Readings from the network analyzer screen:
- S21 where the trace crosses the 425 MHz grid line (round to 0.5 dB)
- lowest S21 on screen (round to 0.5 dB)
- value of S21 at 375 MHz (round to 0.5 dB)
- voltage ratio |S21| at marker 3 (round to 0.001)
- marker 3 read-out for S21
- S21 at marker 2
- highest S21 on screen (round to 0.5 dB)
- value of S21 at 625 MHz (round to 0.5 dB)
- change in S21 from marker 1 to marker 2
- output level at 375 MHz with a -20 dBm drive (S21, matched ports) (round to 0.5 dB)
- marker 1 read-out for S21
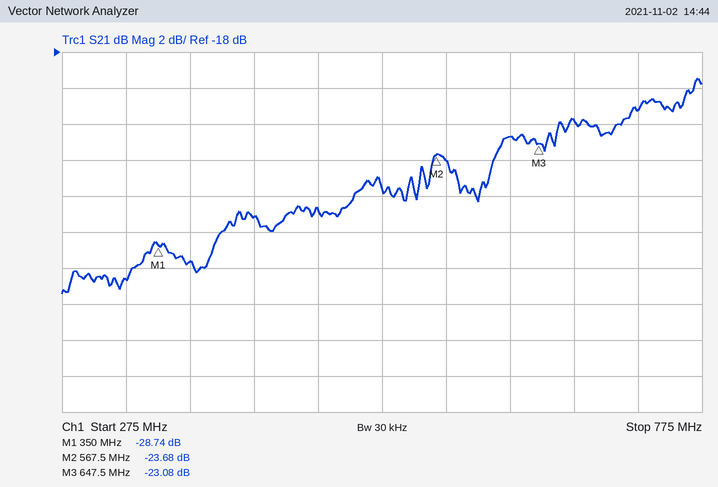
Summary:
-27.0 dB
-31.5 dB
-29.5 dB
0.070
-23.08 dB
-23.68 dB
-19.5 dB
-22.5 dB
5.06 dB
-49.5 dBm
-28.74 dB
